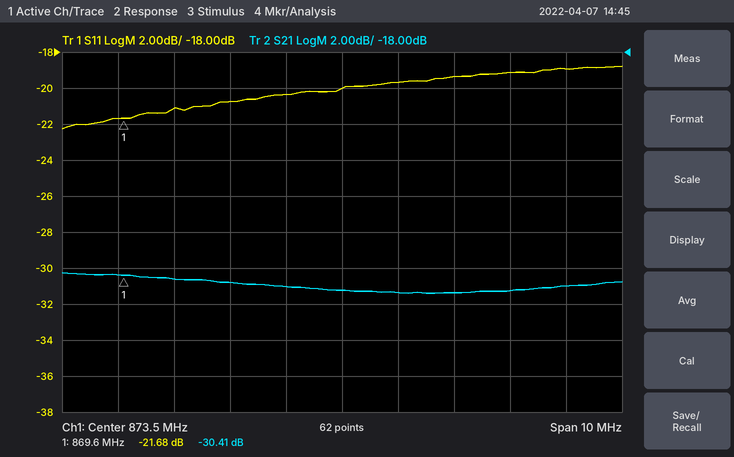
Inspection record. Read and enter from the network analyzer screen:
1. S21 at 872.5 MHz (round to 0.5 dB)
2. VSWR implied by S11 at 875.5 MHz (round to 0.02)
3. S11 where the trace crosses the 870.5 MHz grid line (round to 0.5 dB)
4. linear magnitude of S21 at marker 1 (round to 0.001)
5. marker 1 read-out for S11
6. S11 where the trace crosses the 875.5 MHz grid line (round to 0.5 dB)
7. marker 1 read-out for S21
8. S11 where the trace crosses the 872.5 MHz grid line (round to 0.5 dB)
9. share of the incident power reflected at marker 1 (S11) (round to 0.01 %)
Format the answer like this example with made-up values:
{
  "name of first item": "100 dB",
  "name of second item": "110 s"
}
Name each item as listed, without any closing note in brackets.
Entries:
{
  "S21 at 872.5 MHz": "-31.0 dB",
  "VSWR implied by S11 at 875.5 MHz": "1.24",
  "S11 where the trace crosses the 870.5 MHz grid line": "-21.0 dB",
  "linear magnitude of S21 at marker 1": "0.030",
  "marker 1 read-out for S11": "-21.68 dB",
  "S11 where the trace crosses the 875.5 MHz grid line": "-19.5 dB",
  "marker 1 read-out for S21": "-30.41 dB",
  "S11 where the trace crosses the 872.5 MHz grid line": "-20.5 dB",
  "share of the incident power reflected at marker 1 (S11)": "0.68 %"
}
